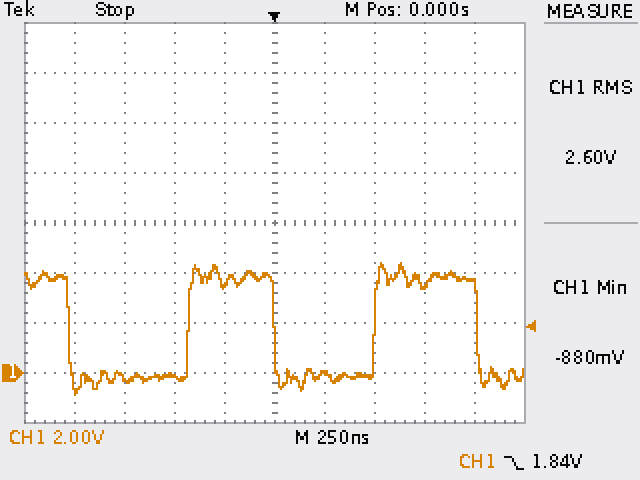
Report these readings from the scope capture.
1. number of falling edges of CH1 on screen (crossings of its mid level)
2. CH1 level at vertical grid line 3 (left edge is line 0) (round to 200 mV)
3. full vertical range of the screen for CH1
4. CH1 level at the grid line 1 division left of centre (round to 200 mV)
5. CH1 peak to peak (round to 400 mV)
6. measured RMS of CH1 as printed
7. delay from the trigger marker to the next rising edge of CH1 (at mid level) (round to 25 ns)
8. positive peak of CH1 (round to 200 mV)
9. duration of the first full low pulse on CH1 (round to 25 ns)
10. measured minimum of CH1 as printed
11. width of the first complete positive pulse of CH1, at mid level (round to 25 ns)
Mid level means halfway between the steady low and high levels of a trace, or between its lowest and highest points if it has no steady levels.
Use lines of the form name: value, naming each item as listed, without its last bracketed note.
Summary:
number of falling edges of CH1 on screen: 3
CH1 level at vertical grid line 3 (left edge is line 0): -200 mV
full vertical range of the screen for CH1: 16 V
CH1 level at the grid line 1 division left of centre: 3.6 V
CH1 peak to peak: 5.2 V
measured RMS of CH1 as printed: 2.60 V
delay from the trigger marker to the next rising edge of CH1 (at mid level): 500 ns
positive peak of CH1: 4.4 V
duration of the first full low pulse on CH1: 600 ns
measured minimum of CH1 as printed: -880 mV
width of the first complete positive pulse of CH1, at mid level: 425 ns
